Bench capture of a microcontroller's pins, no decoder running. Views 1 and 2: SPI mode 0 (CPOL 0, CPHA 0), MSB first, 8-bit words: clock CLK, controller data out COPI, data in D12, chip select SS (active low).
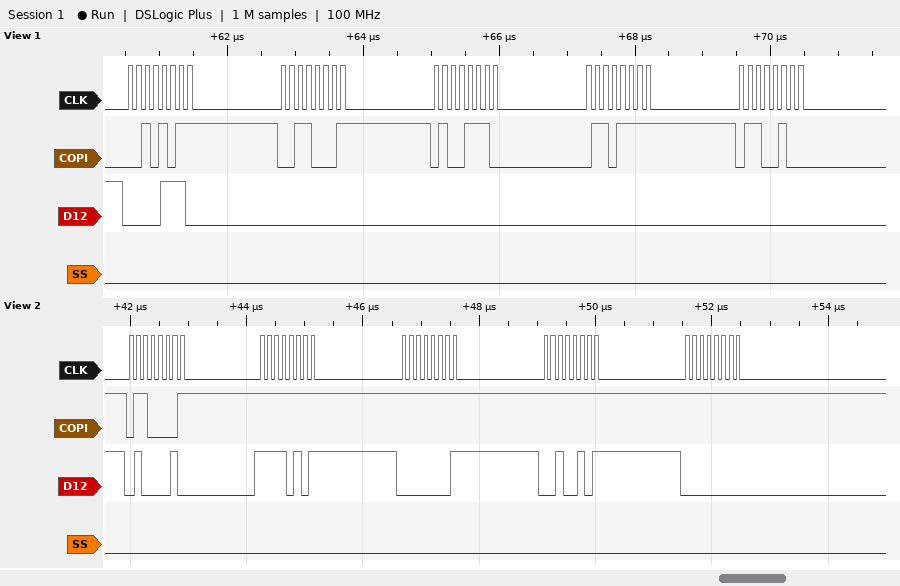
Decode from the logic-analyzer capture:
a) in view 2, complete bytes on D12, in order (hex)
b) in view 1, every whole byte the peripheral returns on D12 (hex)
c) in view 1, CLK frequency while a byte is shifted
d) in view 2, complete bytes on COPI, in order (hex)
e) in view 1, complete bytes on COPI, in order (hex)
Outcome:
42 F5 01 25 00
0x0E 0x00 0x00 0x00 0x00
8 MHz
61 FF FF FF FF
0x2B 0x31 0x4E 0x6F 0x64
